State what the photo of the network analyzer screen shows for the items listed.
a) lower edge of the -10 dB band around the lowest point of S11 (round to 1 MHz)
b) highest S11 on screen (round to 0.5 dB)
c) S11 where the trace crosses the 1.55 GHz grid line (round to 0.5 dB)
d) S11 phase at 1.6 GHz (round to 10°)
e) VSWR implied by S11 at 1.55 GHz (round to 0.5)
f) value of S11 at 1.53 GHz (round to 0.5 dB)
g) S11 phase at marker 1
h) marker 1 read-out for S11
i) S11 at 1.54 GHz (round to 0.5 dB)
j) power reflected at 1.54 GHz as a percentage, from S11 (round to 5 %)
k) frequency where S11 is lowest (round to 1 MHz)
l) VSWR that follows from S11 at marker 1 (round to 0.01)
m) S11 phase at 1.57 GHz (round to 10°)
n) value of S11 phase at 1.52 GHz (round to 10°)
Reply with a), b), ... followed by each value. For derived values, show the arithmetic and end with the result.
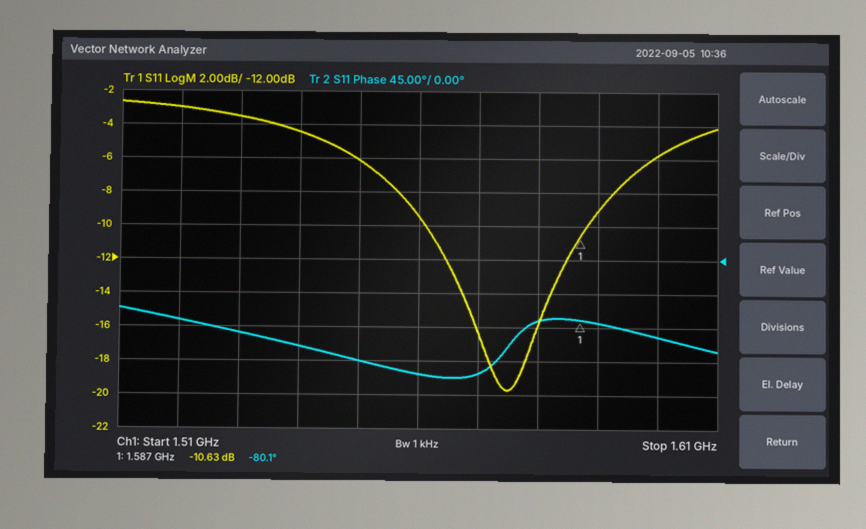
a) 1.561 GHz
b) -2.5 dB
c) -6.0 dB
d) -100°
e) |Γ| = 10^(-6/20) = 0.5012; VSWR = (1 + 0.5012)/(1 − 0.5012) ≈ 3.0
f) -3.5 dB
g) -80.1°
h) -10.63 dB
i) -4.5 dB
j) 10^(-4.5/10) ≈ 35 %
k) 1.575 GHz
l) (1 + 0.2941)/(1 − 0.2941) ≈ 1.83
m) -150°
n) -80°
